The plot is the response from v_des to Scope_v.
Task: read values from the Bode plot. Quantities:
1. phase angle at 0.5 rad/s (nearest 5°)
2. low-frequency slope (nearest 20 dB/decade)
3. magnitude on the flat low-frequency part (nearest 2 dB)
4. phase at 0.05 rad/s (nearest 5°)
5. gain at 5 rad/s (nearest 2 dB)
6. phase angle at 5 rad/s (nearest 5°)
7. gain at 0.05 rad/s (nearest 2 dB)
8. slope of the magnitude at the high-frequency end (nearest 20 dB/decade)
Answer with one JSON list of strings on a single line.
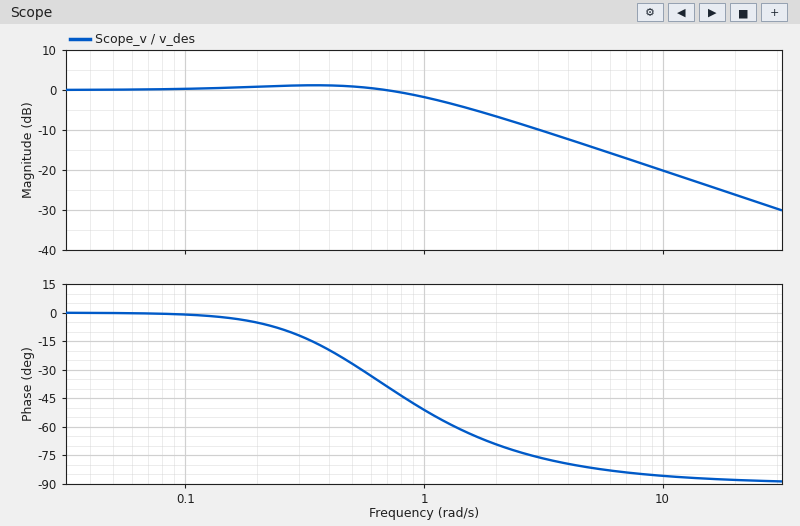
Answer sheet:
["-25°", "0 dB/decade", "0 dB", "0°", "-14 dB", "-80°", "0 dB", "-20 dB/decade"]
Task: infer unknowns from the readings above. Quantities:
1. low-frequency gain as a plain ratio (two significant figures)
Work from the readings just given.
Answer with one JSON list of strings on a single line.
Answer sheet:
["1.0"]
